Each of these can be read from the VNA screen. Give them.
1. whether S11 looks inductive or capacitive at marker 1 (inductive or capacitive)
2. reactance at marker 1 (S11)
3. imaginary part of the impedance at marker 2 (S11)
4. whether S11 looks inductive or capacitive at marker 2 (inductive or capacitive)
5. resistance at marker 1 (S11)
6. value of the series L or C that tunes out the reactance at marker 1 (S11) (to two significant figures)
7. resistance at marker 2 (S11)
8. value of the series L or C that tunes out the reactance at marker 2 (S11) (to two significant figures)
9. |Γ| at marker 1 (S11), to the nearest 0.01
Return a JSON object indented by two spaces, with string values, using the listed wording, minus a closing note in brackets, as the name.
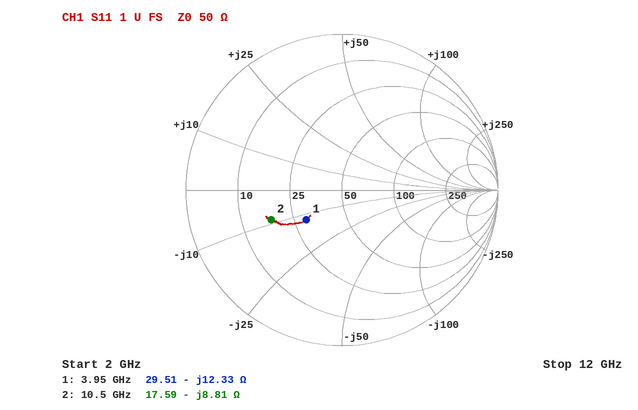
{
  "whether S11 looks inductive or capacitive at marker 1": "capacitive",
  "reactance at marker 1": "-12.33 Ω",
  "imaginary part of the impedance at marker 2": "-8.81 Ω",
  "whether S11 looks inductive or capacitive at marker 2": "capacitive",
  "resistance at marker 1": "29.51 Ω",
  "value of the series L or C that tunes out the reactance at marker 1 (S11)": "500 pH",
  "resistance at marker 2": "17.59 Ω",
  "value of the series L or C that tunes out the reactance at marker 2 (S11)": "130 pH",
  "|Γ| at marker 1 (S11), to the nearest 0.01": "0.30"
}
